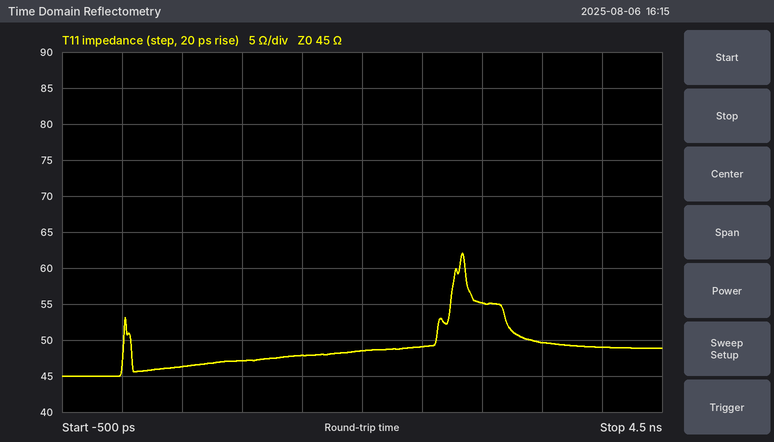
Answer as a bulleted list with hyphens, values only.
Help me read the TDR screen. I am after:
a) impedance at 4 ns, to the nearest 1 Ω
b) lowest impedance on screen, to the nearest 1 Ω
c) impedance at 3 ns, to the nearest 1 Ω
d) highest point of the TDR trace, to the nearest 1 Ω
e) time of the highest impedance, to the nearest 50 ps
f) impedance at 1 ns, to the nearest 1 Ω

- 49 Ω
- 45 Ω
- 55 Ω
- 62 Ω
- 2.85 ns
- 47 Ω
